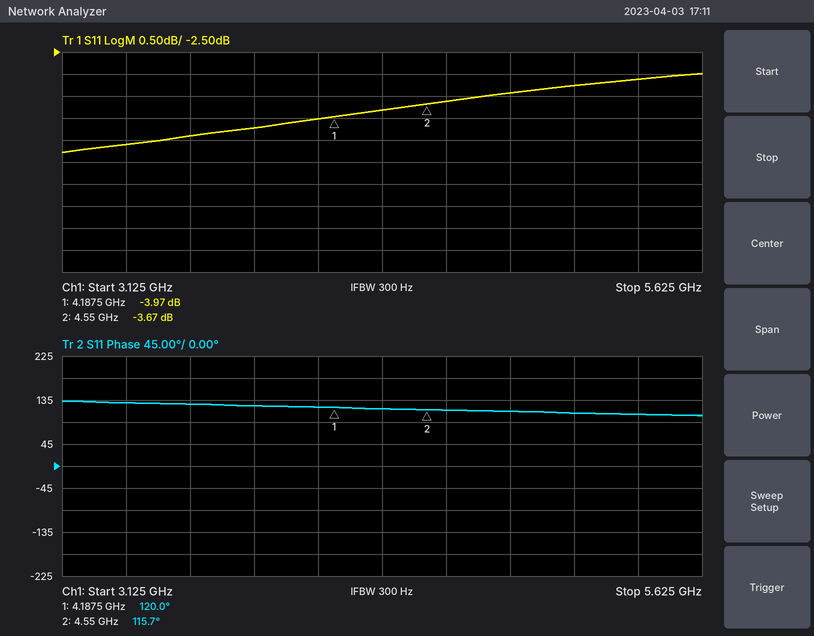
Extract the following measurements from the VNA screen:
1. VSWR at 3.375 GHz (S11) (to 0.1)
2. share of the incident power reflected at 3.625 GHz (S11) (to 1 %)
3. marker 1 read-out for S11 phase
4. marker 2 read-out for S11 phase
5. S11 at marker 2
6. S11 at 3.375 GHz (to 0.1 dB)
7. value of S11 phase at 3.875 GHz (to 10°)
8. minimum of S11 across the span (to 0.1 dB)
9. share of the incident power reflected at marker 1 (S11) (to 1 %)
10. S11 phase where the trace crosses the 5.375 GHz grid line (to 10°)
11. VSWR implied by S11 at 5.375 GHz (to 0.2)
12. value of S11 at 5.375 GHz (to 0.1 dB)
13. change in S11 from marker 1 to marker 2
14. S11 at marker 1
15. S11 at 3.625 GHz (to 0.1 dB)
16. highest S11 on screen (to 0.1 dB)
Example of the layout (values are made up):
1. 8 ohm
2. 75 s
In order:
1. 3.9
2. 36 %
3. 120.0°
4. 115.7°
5. -3.67 dB
6. -4.6 dB
7. 120°
8. -4.8 dB
9. 40 %
10. 110°
11. 5.6
12. -3.1 dB
13. 0.30 dB
14. -3.97 dB
15. -4.4 dB
16. -3.0 dB
